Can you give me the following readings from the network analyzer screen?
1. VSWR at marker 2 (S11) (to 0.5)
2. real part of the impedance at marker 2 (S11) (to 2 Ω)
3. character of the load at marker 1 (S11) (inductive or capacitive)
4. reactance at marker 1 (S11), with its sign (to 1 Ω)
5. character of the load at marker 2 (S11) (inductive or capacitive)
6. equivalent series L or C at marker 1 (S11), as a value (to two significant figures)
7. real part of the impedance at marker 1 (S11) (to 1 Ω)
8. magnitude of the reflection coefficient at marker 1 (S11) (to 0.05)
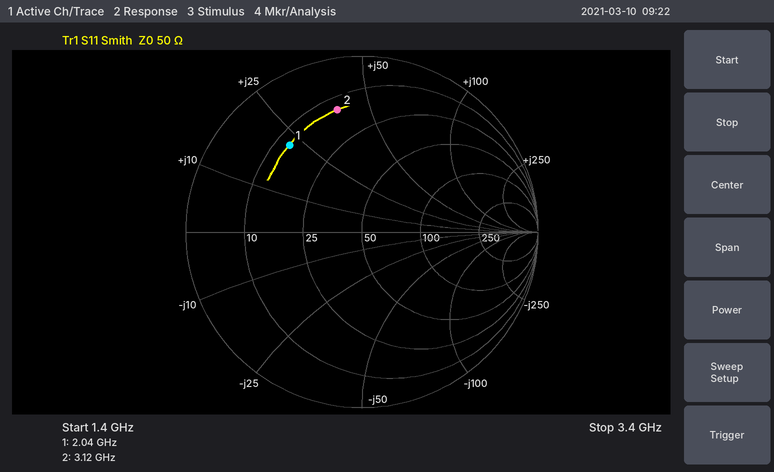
6.0
14 Ω
inductive
+22 Ω
inductive
1.7 nH
13 Ω
0.65
